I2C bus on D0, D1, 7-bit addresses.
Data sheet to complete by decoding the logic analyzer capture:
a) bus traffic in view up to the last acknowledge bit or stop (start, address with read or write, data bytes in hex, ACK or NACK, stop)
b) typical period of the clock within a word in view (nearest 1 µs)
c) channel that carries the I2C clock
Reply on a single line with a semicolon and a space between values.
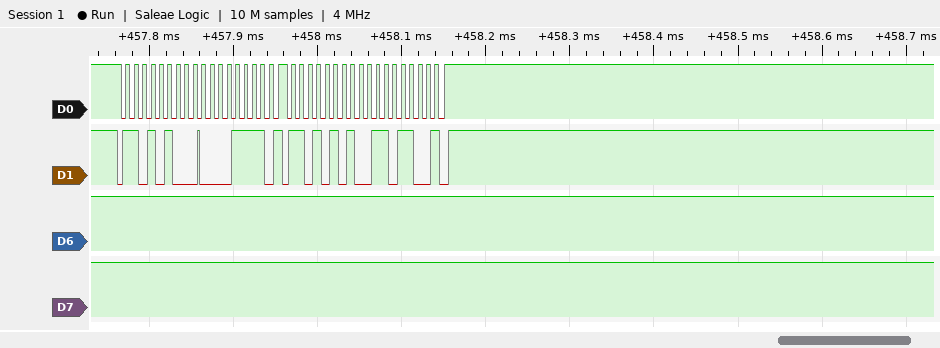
start, address 6A write ACK, 0F ACK, repeated start, address 6A read ACK, 6C NACK, stop; 10 µs; D0
